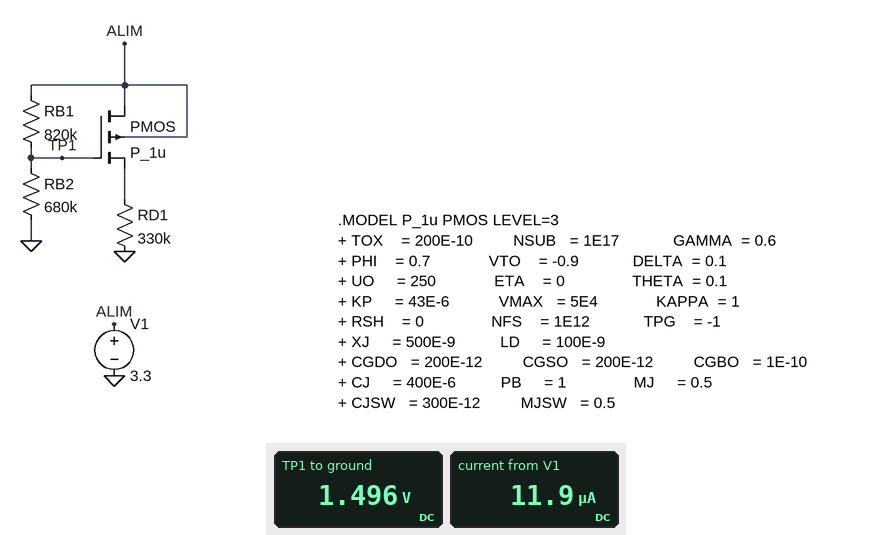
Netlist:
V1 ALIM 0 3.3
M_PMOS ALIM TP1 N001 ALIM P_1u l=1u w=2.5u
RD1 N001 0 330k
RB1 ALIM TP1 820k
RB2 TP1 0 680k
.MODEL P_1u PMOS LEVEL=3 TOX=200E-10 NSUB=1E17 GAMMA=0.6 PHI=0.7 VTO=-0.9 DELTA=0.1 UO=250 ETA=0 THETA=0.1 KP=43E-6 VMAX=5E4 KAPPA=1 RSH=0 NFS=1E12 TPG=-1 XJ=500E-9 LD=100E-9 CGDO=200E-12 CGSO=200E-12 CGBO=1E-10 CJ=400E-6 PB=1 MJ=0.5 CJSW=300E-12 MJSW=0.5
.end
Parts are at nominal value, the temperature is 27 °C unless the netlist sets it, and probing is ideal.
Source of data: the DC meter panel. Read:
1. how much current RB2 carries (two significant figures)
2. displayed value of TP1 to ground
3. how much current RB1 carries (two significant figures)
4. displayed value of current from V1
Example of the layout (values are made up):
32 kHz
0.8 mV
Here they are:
2.2 µA
1.496 V
2.2 µA
11.9 µA
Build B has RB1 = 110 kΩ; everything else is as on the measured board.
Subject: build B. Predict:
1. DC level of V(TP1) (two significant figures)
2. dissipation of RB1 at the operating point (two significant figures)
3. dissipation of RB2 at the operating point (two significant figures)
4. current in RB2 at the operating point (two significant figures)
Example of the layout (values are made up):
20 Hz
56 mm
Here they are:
2.8 V
1.9 µW
12 µW
4.2 µA
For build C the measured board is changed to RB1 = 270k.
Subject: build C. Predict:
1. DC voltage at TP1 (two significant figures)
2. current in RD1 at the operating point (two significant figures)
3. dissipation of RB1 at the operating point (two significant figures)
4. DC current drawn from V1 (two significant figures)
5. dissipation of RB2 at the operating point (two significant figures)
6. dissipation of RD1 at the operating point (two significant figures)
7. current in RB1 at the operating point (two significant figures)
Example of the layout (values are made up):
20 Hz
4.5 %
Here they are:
2.4 V
610 nA
3.3 µW
4.1 µA
8.2 µW
120 nW
3.5 µA
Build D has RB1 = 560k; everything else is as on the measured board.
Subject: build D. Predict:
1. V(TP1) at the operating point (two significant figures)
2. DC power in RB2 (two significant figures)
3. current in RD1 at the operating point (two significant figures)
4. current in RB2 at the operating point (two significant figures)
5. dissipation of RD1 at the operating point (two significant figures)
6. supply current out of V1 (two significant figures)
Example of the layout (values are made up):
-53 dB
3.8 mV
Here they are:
1.8 V
4.8 µW
9.6 µA
2.7 µA
30 µW
12 µA
